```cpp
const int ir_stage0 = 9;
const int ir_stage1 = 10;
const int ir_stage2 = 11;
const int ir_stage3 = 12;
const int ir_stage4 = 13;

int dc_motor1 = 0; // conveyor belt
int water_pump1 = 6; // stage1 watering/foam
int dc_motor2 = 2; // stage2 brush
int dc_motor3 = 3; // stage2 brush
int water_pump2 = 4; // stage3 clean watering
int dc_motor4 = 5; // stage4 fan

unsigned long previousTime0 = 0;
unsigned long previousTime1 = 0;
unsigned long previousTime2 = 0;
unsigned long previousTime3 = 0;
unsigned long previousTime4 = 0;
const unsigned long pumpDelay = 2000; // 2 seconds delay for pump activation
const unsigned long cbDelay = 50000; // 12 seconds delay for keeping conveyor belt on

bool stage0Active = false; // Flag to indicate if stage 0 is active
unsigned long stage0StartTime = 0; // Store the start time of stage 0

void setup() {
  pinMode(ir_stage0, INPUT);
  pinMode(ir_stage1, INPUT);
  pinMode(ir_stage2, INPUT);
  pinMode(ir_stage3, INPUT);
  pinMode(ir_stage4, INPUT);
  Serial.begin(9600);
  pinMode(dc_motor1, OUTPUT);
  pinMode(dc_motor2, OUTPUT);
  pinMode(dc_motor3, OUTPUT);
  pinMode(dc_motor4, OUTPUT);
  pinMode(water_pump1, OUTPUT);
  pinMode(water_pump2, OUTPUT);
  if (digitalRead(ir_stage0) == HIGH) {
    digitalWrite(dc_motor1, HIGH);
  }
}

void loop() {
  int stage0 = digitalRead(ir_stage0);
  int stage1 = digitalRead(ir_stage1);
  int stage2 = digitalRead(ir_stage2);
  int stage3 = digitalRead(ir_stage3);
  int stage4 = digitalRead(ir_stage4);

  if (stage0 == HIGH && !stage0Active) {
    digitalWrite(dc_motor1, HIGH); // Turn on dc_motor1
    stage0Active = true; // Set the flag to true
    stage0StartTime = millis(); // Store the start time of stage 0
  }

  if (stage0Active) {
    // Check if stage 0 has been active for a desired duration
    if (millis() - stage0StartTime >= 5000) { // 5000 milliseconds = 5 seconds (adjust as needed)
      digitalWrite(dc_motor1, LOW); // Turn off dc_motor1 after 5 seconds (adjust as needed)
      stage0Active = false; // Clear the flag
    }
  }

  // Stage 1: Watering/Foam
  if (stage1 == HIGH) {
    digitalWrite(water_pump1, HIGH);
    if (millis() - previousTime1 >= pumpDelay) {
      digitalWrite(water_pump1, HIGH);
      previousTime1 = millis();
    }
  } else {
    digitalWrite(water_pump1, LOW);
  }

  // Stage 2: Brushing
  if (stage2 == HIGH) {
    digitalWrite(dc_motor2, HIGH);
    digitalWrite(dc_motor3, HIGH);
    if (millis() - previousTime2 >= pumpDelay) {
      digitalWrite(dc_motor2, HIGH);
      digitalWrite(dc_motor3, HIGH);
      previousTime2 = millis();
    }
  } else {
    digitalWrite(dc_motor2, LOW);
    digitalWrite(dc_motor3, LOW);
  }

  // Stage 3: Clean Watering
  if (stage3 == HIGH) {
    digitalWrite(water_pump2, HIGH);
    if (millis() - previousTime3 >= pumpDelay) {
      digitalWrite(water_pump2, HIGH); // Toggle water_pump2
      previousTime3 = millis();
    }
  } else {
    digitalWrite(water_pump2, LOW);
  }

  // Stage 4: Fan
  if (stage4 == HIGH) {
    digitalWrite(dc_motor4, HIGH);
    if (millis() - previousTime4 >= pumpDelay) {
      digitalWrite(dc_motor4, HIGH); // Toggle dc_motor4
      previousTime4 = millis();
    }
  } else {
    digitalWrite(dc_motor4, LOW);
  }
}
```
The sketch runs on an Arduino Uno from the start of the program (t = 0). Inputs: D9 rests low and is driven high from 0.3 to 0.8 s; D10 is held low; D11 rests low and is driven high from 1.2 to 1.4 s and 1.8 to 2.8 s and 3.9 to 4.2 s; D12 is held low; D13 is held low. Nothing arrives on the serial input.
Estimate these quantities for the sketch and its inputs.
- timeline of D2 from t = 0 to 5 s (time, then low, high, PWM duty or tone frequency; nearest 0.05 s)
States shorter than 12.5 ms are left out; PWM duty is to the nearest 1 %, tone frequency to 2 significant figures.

0 s low; 1.2 s high; 1.4 s low; 1.8 s high; 2.8 s low; 3.9 s high; 4.2 s low
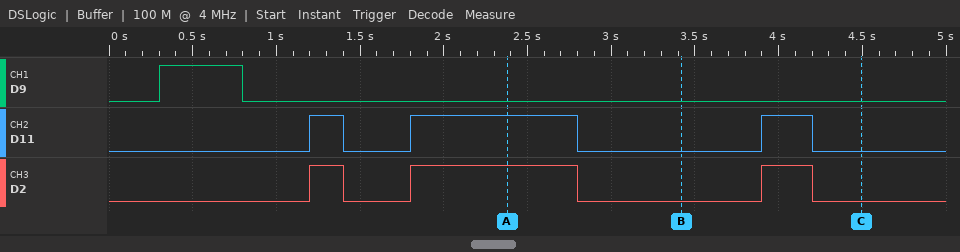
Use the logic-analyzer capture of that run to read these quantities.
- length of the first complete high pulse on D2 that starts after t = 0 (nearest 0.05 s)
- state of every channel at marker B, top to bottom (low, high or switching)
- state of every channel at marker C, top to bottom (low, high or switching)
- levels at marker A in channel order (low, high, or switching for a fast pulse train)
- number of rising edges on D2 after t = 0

0.20 s
D9 low, D11 low, D2 low
D9 low, D11 low, D2 low
D9 low, D11 high, D2 high
3
